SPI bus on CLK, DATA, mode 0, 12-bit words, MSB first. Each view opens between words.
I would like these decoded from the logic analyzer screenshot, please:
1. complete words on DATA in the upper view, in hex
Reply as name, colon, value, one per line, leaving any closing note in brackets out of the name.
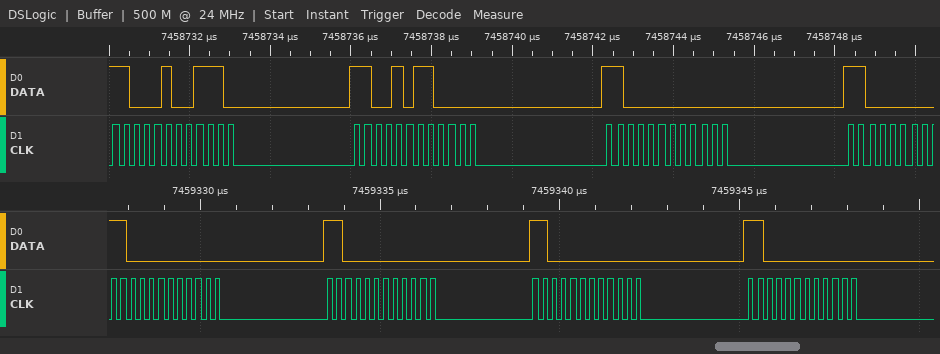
complete words on DATA in the upper view, in hex: C4E, CB0, C00
